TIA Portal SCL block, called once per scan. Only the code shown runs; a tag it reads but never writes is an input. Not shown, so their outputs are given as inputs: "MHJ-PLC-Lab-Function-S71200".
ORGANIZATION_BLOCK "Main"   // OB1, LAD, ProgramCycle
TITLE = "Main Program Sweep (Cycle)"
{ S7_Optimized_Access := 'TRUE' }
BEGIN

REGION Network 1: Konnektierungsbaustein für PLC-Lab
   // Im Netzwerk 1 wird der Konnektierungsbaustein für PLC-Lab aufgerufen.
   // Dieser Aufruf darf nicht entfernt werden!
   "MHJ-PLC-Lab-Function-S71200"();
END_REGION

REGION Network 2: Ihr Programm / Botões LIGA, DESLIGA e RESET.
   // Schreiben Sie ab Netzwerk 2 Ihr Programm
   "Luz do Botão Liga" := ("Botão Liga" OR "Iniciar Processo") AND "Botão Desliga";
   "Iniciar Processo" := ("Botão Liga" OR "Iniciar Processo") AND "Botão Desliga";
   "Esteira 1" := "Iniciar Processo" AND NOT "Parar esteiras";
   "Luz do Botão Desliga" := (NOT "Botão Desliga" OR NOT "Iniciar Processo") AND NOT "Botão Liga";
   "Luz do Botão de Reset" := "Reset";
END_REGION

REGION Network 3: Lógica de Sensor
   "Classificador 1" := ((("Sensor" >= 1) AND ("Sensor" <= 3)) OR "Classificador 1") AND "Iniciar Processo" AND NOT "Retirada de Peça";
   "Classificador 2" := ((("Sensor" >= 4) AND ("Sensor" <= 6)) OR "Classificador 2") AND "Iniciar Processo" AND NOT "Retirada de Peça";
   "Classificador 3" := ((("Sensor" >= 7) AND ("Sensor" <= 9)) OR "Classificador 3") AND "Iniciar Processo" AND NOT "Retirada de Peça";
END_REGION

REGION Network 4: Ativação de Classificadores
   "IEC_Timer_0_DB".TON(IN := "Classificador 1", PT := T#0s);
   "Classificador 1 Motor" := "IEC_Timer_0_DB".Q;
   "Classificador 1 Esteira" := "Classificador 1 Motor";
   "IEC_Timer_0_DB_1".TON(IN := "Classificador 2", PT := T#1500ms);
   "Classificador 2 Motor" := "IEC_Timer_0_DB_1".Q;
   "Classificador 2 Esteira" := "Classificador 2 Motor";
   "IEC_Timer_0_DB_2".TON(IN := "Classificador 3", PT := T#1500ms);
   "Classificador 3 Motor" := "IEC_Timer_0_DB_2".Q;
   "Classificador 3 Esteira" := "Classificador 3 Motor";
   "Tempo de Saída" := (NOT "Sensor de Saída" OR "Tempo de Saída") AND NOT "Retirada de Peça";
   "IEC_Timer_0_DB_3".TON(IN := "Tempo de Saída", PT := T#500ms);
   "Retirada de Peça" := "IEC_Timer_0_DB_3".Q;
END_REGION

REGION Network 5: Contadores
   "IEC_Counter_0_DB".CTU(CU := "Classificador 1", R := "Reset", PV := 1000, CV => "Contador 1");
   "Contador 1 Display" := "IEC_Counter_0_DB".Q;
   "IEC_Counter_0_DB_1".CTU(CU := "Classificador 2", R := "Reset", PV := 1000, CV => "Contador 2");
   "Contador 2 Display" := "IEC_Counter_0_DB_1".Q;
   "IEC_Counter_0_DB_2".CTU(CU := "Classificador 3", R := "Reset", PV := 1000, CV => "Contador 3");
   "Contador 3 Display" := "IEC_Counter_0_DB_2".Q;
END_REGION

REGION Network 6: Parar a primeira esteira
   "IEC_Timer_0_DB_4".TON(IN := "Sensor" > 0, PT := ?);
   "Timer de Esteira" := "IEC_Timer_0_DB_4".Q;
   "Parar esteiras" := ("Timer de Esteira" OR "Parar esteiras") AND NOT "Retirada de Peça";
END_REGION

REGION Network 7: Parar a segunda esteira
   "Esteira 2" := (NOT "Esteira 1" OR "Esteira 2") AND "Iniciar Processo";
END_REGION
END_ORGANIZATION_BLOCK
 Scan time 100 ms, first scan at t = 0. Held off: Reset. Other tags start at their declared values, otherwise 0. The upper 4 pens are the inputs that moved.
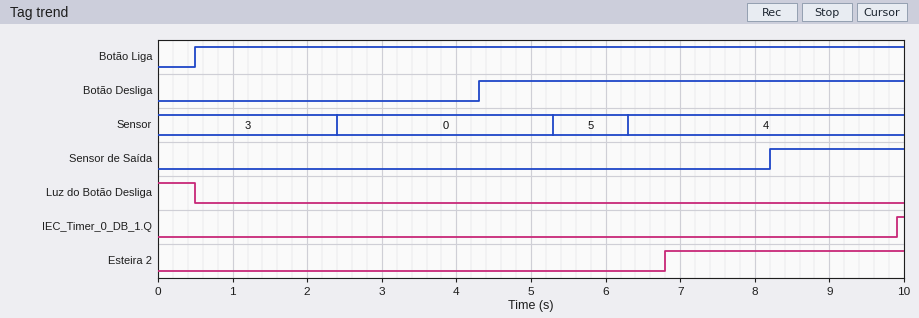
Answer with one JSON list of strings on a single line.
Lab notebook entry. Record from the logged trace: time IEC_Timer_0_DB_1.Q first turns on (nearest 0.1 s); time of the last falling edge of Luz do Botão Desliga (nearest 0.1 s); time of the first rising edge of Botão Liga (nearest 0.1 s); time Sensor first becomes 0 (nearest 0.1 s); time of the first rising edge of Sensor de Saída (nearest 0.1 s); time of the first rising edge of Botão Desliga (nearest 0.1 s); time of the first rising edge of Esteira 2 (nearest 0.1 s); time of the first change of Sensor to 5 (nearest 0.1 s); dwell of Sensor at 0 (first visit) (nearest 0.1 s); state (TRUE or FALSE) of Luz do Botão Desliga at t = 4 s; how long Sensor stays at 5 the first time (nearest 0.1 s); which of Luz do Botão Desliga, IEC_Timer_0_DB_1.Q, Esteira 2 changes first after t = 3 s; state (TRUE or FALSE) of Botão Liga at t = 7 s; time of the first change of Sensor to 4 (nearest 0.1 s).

["9.9 s", "0.5 s", "0.5 s", "2.4 s", "8.2 s", "4.3 s", "6.8 s", "5.3 s", "2.9 s", "FALSE", "1.0 s", "Esteira 2", "TRUE", "6.3 s"]
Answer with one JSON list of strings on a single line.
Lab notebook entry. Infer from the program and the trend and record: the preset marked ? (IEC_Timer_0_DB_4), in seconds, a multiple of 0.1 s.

["1.4 s"]
